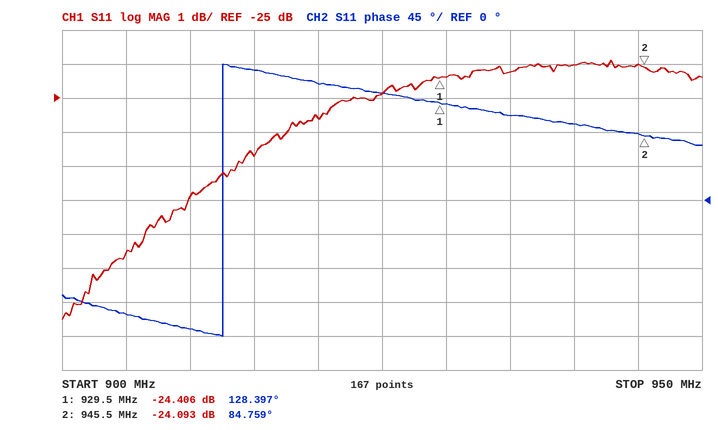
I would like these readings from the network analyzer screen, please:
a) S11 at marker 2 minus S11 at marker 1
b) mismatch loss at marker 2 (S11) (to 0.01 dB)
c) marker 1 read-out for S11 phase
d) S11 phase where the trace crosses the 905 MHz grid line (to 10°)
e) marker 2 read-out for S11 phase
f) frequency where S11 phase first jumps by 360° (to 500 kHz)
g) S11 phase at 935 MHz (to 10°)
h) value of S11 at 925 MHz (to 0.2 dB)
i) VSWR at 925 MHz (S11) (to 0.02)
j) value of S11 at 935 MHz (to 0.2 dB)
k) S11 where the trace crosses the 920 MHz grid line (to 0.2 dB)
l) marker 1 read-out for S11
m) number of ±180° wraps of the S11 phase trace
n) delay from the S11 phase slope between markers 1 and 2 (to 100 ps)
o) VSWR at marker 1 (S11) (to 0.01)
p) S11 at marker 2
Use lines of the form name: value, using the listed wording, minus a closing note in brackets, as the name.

S11 at marker 2 minus S11 at marker 1: 0.313 dB
mismatch loss at marker 2 (S11): 0.02 dB
marker 1 read-out for S11 phase: 128.397°
S11 phase where the trace crosses the 905 MHz grid line: -150°
marker 2 read-out for S11 phase: 84.759°
frequency where S11 phase first jumps by 360°: 912.5 MHz
S11 phase at 935 MHz: 110°
value of S11 at 925 MHz: -24.8 dB
VSWR at 925 MHz (S11): 1.12
value of S11 at 935 MHz: -24.2 dB
S11 where the trace crosses the 920 MHz grid line: -25.6 dB
marker 1 read-out for S11: -24.406 dB
number of ±180° wraps of the S11 phase trace: 1
delay from the S11 phase slope between markers 1 and 2: 7.6 ns
VSWR at marker 1 (S11): 1.13
S11 at marker 2: -24.093 dB
